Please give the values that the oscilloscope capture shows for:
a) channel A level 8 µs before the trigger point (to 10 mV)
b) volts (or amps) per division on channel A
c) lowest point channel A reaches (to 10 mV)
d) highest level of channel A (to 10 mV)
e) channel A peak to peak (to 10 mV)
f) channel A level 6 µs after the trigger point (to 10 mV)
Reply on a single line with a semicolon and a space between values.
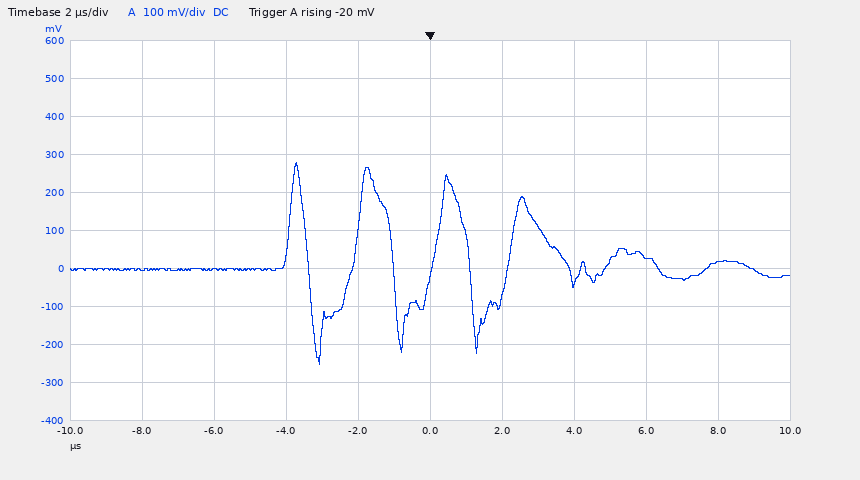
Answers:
0 mV; 100 mV; -250 mV; 280 mV; 530 mV; 30 mV
